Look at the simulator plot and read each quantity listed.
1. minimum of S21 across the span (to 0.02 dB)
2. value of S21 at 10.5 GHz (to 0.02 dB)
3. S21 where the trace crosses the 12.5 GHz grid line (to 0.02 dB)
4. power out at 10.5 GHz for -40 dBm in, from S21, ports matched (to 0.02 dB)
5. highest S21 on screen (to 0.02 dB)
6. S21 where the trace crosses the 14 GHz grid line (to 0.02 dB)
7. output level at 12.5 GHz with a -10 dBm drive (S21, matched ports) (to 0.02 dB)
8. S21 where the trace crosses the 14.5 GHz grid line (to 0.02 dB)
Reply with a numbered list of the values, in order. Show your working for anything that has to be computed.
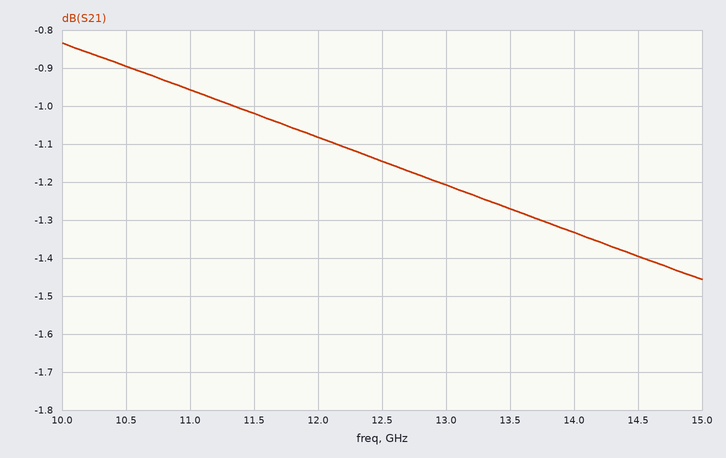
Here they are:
1. -1.46 dB
2. -0.90 dB
3. -1.14 dB
4. -40 dBm + (-0.90 dB) = -40.90 dBm
5. -0.84 dB
6. -1.34 dB
7. -10 dBm + (-1.14 dB) = -11.14 dBm
8. -1.40 dB
